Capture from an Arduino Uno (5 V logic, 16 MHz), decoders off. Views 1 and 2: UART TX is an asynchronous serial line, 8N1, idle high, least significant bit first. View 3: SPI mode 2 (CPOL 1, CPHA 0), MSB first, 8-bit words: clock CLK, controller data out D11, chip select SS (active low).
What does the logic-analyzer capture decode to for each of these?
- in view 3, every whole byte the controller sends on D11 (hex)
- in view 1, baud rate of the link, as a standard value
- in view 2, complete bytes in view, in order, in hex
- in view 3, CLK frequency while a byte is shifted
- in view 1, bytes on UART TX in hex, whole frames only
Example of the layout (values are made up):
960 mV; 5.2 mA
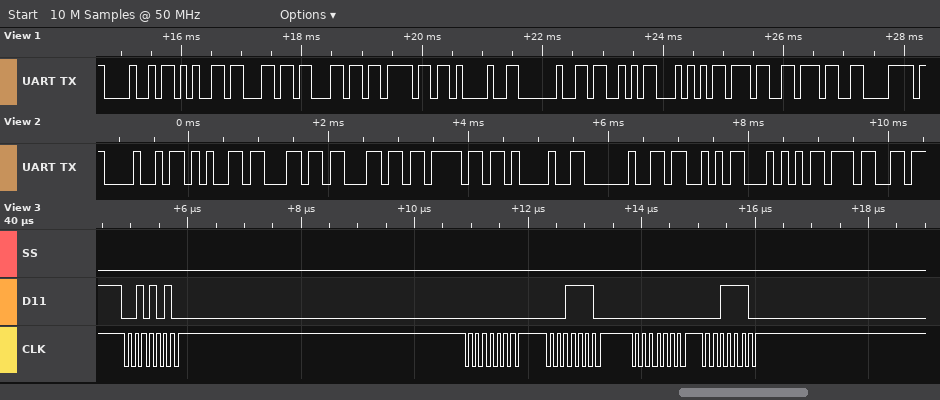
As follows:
2A 00 1E 00 1E; 9600 baud; 48 65 6C 6C 6F 21 20 53 54 37; 8 MHz; 48 65 6C 6C 6F 21 20 53 54 37 37 78
